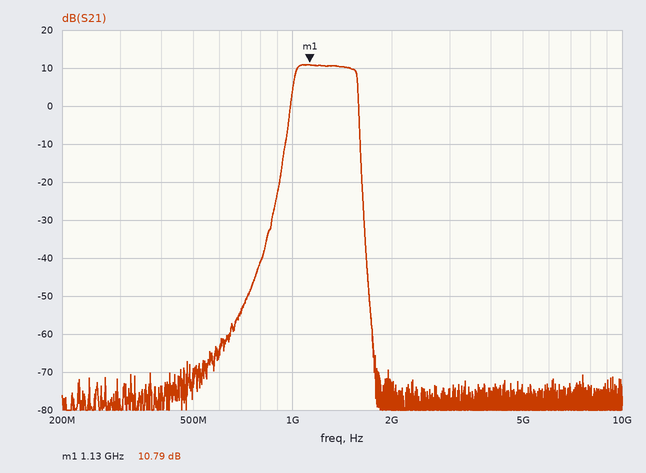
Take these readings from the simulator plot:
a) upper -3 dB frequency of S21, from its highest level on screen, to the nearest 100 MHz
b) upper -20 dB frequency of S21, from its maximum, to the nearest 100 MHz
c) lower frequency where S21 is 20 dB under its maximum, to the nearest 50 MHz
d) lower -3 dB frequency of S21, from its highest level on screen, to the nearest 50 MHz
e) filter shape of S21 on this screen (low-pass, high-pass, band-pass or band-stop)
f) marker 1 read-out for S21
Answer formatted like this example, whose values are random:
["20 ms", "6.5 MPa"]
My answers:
["1.6 GHz", "1.6 GHz", "950 MHz", "1.00 GHz", "band-pass", "10.79 dB"]
